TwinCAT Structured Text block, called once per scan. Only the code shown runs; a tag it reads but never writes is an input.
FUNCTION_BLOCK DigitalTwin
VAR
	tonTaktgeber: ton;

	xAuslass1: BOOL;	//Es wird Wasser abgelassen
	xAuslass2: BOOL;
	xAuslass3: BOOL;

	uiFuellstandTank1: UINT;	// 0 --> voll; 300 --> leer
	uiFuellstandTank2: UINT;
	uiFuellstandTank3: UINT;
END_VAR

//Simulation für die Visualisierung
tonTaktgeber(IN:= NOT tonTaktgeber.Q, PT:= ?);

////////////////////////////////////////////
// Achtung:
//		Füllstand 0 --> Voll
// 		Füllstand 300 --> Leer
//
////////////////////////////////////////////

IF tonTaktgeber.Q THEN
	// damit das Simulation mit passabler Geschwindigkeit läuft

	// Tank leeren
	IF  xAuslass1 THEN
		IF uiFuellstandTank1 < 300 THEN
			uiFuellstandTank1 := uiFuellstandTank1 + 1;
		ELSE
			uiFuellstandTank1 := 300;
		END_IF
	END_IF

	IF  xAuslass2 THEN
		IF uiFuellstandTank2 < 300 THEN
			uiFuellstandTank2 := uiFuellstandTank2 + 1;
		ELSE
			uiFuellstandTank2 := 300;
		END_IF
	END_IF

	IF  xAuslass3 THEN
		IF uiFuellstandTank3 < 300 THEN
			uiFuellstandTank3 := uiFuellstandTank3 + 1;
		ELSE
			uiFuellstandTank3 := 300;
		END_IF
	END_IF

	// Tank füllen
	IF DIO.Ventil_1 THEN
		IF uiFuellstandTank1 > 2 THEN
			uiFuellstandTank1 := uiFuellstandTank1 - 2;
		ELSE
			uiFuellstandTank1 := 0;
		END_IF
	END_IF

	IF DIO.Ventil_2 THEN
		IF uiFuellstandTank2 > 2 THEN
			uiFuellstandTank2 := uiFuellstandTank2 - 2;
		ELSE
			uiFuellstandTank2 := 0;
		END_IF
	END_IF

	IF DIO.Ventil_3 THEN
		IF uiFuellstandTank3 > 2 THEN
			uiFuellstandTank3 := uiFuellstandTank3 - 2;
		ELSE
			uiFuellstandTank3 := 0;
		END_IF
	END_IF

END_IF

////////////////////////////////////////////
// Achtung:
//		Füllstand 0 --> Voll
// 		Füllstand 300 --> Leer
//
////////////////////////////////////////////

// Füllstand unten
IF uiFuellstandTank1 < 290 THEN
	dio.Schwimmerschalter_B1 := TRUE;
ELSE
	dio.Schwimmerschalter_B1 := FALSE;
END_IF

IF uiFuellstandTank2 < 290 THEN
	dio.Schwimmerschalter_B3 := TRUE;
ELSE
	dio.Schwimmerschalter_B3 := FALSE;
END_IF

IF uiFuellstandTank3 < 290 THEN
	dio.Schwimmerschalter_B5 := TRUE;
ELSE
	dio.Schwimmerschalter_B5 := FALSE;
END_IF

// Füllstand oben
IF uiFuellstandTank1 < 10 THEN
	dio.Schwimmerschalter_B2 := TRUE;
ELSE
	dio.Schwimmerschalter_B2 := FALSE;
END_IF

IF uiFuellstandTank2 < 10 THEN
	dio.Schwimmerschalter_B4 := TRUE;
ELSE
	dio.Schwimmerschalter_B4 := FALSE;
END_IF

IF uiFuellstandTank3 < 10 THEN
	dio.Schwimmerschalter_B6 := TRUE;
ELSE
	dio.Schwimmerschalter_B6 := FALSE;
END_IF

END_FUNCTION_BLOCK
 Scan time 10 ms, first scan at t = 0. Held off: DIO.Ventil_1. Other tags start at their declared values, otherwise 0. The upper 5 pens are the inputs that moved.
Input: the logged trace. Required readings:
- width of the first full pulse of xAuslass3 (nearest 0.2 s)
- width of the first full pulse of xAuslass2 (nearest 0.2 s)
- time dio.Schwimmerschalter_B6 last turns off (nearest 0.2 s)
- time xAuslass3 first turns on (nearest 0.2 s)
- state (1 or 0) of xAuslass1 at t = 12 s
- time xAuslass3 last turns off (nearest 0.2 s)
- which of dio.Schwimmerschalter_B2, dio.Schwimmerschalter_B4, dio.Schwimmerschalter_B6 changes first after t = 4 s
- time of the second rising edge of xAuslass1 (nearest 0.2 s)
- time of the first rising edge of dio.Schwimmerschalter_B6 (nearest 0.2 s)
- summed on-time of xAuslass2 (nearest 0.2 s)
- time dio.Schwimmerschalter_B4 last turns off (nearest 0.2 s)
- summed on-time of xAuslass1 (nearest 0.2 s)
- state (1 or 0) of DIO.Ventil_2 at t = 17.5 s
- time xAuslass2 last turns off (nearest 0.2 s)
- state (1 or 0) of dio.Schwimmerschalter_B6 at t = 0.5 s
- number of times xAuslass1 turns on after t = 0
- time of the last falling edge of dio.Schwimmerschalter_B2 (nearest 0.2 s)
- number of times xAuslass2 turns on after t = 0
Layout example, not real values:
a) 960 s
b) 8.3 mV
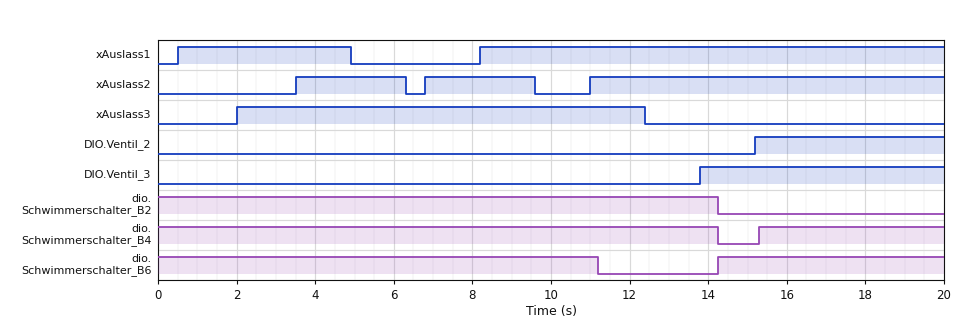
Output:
a) 10.4 s
b) 2.8 s
c) 11.2 s
d) 2.0 s
e) 1
f) 12.4 s
g) dio.Schwimmerschalter_B6
h) 8.2 s
i) 14.2 s
j) 14.6 s
k) 14.2 s
l) 16.2 s
m) 1
n) 9.6 s
o) 1
p) 2
q) 14.2 s
r) 3
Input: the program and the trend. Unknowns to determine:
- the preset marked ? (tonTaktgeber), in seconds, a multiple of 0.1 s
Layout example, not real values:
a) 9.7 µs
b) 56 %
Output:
a) 1.0 s
